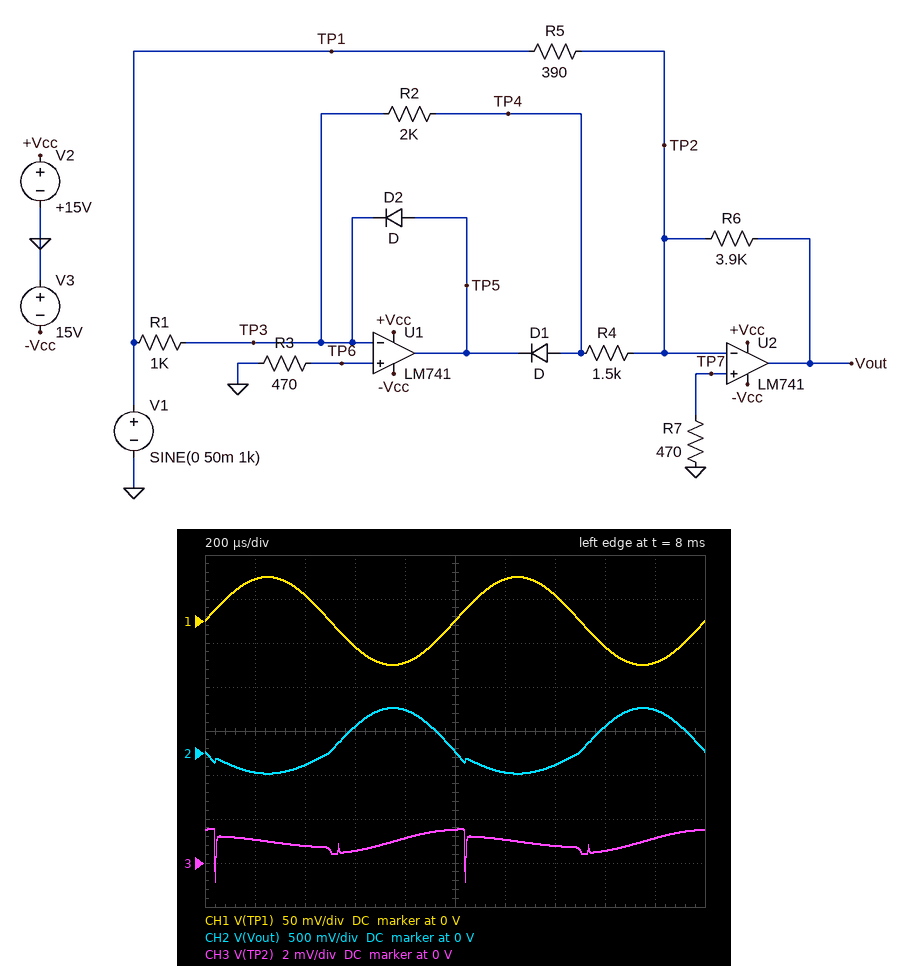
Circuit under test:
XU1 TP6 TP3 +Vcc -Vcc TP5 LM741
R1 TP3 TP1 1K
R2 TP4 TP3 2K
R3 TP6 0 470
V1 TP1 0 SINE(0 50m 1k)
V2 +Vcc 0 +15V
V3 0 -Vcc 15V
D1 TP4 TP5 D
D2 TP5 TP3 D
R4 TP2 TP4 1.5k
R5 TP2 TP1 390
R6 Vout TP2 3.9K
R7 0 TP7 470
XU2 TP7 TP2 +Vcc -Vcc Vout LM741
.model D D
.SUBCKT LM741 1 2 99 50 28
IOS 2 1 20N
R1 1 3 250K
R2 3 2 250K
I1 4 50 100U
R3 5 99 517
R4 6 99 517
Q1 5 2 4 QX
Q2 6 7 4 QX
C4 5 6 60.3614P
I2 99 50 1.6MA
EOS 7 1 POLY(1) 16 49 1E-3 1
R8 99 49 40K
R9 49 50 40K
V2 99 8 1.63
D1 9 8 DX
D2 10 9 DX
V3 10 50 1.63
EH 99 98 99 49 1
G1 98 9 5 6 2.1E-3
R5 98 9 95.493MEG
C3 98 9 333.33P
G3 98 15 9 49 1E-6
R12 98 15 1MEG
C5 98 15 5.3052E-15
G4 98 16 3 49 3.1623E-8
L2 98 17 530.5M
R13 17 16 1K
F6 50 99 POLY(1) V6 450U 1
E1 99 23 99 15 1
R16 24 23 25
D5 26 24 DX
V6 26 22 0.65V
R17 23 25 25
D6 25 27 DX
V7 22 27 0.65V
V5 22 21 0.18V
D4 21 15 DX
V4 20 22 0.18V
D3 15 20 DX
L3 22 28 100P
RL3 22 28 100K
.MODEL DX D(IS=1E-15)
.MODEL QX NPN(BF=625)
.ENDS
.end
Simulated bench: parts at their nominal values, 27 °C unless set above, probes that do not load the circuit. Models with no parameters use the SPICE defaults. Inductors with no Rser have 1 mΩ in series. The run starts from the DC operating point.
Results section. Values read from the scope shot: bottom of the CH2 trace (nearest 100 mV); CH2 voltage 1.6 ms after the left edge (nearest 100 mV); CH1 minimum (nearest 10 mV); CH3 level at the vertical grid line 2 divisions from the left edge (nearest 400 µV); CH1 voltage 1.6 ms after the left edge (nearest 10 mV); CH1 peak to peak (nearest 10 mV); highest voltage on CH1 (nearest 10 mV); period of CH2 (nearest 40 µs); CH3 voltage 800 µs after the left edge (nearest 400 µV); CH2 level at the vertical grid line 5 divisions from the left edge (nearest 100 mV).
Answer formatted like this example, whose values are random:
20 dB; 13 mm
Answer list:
-200 mV; 300 mV; -50 mV; 800 µV; -30 mV; 100 mV; 50 mV; 1.00 ms; 1.2 mV; 0 V
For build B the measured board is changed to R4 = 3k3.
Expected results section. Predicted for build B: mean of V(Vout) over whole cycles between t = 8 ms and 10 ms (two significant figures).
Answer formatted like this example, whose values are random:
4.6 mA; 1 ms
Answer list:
47 mV
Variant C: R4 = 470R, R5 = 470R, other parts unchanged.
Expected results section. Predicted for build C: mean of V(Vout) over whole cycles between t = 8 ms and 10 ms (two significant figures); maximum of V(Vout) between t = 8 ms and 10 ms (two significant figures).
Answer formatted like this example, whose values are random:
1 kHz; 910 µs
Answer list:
260 mV; 420 mV
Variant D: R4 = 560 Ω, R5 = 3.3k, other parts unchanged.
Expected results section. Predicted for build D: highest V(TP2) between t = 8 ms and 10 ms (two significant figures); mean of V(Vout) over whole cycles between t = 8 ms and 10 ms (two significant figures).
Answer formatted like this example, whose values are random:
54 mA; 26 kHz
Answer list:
1.7 mV; 210 mV
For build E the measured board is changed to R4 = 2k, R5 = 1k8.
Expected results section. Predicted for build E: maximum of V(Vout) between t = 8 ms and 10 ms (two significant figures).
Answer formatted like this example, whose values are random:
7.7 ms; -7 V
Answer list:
110 mV
